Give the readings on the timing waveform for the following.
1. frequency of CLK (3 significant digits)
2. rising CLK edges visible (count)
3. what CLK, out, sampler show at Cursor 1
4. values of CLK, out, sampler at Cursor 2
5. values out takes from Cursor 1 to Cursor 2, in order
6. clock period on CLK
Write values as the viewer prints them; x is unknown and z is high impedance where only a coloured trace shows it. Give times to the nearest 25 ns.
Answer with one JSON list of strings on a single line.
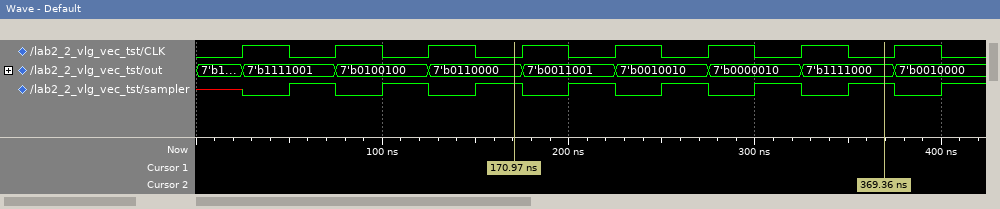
["20.0 MHz", "8", "CLK=0, out=7'b0110000, sampler=1", "CLK=0, out=7'b1111000, sampler=1", "7'b0110000, 7'b0011001, 7'b0010010, 7'b0000010, 7'b1111000", "50 ns"]
